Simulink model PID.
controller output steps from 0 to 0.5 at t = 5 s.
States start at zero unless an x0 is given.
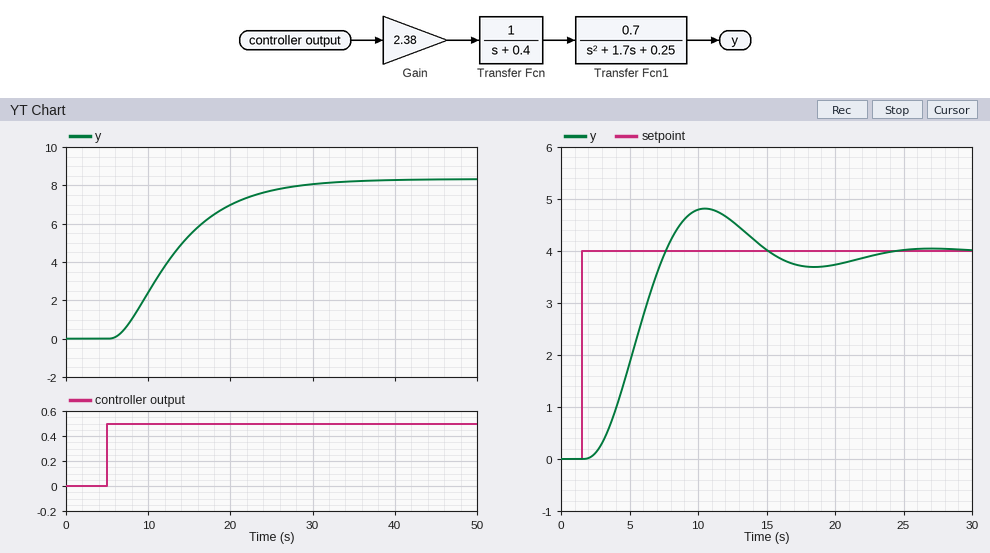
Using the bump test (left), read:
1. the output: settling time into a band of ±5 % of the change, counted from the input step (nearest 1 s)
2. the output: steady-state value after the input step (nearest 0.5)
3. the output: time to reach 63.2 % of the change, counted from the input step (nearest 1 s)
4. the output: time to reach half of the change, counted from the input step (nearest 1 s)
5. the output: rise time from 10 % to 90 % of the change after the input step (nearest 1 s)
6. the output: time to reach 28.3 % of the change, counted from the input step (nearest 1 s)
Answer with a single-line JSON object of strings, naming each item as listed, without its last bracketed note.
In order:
{"the output: settling time into a band of ±5 % of the change, counted from the input step": "22 s", "the output: steady-state value after the input step": "8.5", "the output: time to reach 63.2 % of the change, counted from the input step": "10 s", "the output: time to reach half of the change, counted from the input step": "8 s", "the output: rise time from 10 % to 90 % of the change after the input step": "15 s", "the output: time to reach 28.3 % of the change, counted from the input step": "5 s"}
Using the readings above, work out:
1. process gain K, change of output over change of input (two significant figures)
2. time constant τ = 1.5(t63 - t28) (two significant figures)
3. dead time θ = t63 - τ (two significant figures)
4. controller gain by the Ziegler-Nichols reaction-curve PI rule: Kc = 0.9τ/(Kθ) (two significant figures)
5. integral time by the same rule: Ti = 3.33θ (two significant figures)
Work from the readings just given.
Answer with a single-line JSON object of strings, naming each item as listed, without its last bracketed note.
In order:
{"process gain K, change of output over change of input": "17", "time constant τ = 1.5(t63 - t28)": "7.5 s", "dead time θ = t63 - τ": "2.5 s", "controller gain by the Ziegler-Nichols reaction-curve PI rule: Kc = 0.9τ/(Kθ)": "0.16", "integral time by the same rule: Ti = 3.33θ": "8.3 s"}
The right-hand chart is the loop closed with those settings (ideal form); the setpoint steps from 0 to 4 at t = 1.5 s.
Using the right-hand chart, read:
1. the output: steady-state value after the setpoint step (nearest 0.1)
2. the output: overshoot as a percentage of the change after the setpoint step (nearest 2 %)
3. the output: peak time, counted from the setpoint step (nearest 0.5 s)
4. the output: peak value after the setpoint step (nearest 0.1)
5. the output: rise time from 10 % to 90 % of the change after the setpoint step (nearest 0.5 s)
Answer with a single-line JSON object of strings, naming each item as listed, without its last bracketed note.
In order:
{"the output: steady-state value after the setpoint step": "4.0", "the output: overshoot as a percentage of the change after the setpoint step": "20 %", "the output: peak time, counted from the setpoint step": "9.0 s", "the output: peak value after the setpoint step": "4.8", "the output: rise time from 10 % to 90 % of the change after the setpoint step": "4.0 s"}
